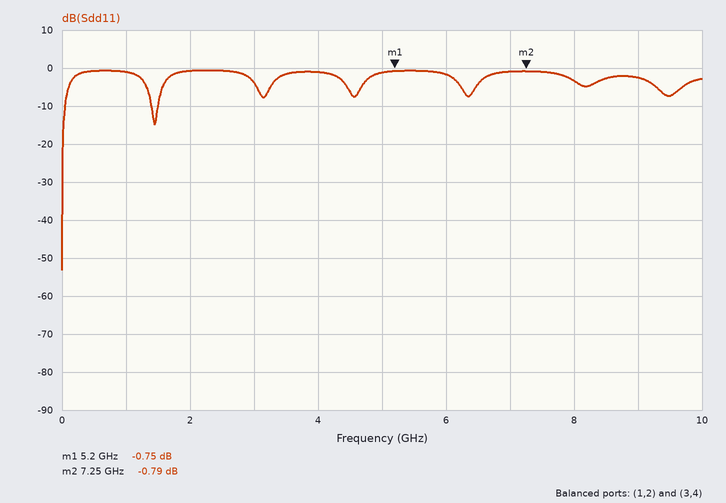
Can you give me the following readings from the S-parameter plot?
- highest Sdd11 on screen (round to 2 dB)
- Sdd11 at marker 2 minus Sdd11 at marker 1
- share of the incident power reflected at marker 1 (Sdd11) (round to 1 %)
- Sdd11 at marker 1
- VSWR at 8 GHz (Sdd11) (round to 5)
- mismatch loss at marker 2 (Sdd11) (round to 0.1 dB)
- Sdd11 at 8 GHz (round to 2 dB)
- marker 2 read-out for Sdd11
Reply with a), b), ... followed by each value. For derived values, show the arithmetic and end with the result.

a) 0 dB
b) -0.79 − (-0.75) = -0.04 dB
c) 10^(-0.75/10) ≈ 84 %
d) -0.75 dB
e) |Γ| = 10^(-4/20) = 0.6310; VSWR = (1 + 0.6310)/(1 − 0.6310) ≈ 4.42, so 5 to the nearest 5
f) −10 log10(1 − 10^(-0.79/10)) ≈ 7.8 dB
g) -4 dB
h) -0.79 dB
